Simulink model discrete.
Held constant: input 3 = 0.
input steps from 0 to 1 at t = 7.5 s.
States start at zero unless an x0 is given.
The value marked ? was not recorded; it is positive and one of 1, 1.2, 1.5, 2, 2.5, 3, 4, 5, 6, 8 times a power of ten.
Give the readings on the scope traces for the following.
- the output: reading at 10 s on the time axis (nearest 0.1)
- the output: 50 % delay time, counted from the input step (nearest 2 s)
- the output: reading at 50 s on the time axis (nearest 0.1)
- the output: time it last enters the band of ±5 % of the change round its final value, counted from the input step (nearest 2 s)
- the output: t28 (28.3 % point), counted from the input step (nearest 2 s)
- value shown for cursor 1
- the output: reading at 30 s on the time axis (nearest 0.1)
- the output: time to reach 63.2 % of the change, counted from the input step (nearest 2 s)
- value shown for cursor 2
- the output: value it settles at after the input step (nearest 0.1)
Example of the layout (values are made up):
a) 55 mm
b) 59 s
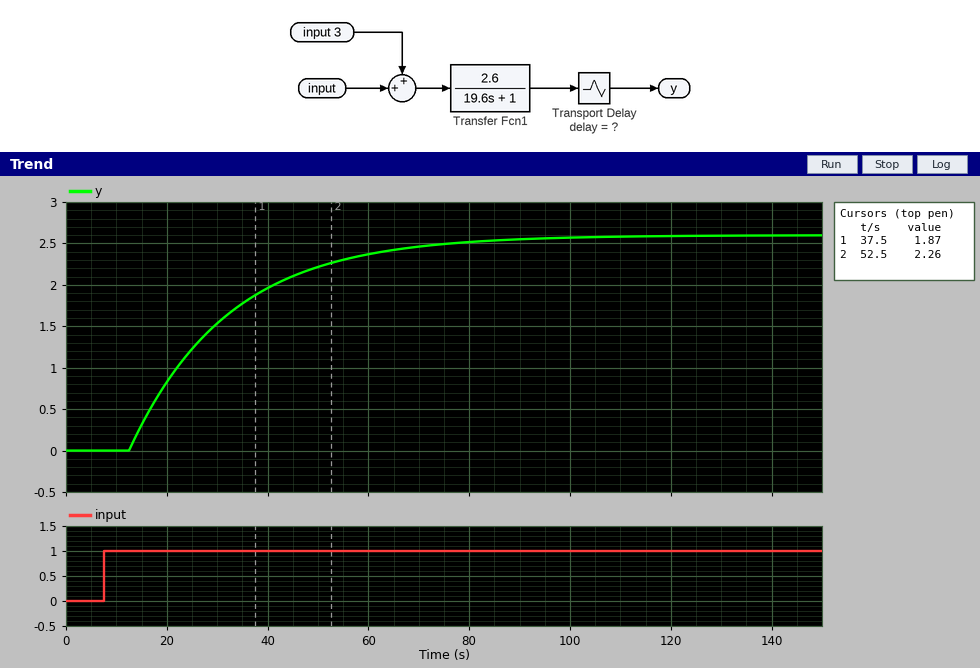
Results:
a) 0.0
b) 18 s
c) 2.2
d) 64 s
e) 12 s
f) 1.87
g) 1.5
h) 24 s
i) 2.26
j) 2.6
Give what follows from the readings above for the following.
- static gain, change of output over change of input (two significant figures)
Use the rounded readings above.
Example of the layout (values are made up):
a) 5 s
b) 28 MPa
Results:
a) 2.6
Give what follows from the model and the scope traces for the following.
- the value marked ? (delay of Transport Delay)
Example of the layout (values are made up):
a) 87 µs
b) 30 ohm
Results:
a) 5
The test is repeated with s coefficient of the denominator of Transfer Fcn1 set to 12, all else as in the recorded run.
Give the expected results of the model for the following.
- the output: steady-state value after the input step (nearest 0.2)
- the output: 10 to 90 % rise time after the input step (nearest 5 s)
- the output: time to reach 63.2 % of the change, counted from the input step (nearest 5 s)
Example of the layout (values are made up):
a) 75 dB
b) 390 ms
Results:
a) 2.6
b) 25 s
c) 15 s
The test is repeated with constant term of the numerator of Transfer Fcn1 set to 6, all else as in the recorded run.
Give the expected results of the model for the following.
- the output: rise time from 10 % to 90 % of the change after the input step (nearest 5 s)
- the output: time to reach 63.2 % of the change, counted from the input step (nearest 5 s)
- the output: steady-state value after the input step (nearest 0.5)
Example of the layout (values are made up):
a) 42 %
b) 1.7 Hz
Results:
a) 45 s
b) 25 s
c) 6.0
